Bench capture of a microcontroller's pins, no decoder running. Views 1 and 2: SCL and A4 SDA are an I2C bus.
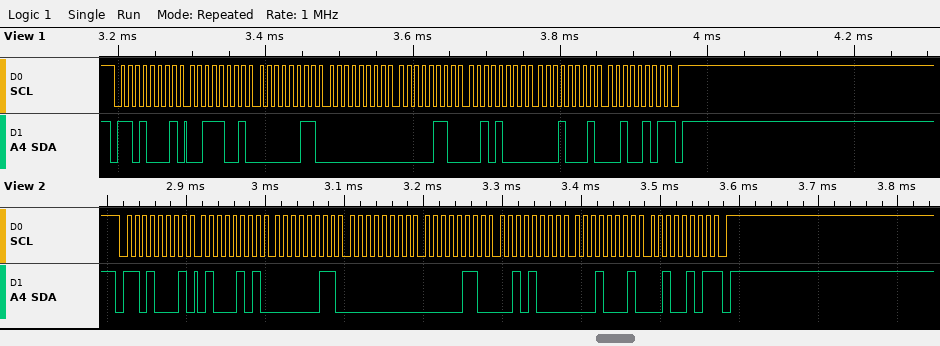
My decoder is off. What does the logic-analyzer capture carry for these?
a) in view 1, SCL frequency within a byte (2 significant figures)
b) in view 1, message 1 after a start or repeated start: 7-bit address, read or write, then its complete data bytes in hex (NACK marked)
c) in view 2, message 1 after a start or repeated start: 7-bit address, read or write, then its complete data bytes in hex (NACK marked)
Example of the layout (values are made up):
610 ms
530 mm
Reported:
100 kHz
0x68 read: 39 03 00 06 28 11 25 NACK
0x68 read: 45 03 00 06 28 11 25 NACK
